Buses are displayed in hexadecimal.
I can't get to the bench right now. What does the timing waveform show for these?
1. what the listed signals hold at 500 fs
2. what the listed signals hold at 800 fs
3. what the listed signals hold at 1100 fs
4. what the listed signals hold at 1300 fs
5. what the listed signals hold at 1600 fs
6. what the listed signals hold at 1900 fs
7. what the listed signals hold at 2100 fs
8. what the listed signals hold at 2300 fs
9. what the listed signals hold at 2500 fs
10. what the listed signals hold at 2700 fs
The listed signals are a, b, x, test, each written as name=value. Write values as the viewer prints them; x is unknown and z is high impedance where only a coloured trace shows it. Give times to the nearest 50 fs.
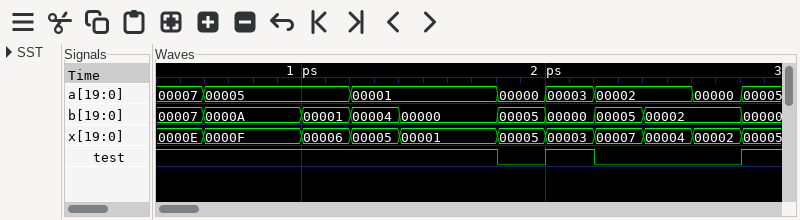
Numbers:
a=00007, b=00007, x=0000E, test=1
a=00005, b=0000A, x=0000F, test=1
a=00005, b=00001, x=00006, test=1
a=00001, b=00004, x=00005, test=1
a=00001, b=00000, x=00001, test=1
a=00000, b=00005, x=00005, test=0
a=00003, b=00000, x=00003, test=1
a=00002, b=00005, x=00007, test=0
a=00002, b=00002, x=00004, test=0
a=00000, b=00002, x=00002, test=0
